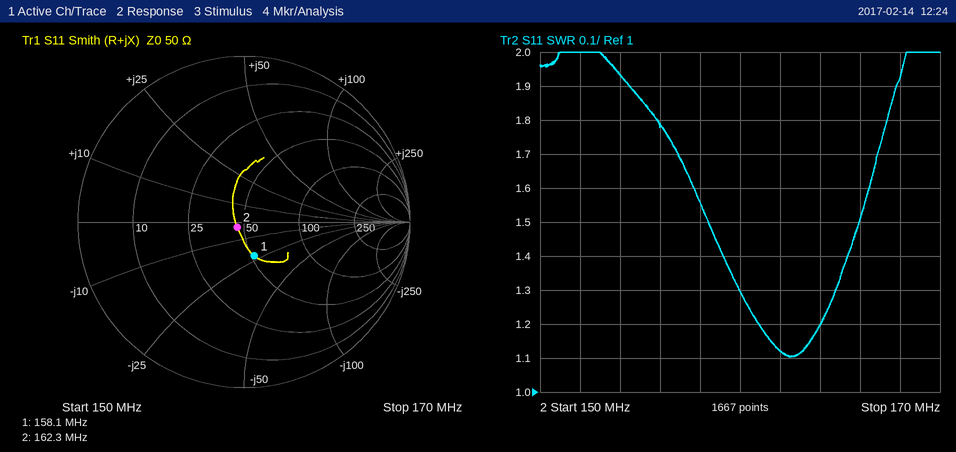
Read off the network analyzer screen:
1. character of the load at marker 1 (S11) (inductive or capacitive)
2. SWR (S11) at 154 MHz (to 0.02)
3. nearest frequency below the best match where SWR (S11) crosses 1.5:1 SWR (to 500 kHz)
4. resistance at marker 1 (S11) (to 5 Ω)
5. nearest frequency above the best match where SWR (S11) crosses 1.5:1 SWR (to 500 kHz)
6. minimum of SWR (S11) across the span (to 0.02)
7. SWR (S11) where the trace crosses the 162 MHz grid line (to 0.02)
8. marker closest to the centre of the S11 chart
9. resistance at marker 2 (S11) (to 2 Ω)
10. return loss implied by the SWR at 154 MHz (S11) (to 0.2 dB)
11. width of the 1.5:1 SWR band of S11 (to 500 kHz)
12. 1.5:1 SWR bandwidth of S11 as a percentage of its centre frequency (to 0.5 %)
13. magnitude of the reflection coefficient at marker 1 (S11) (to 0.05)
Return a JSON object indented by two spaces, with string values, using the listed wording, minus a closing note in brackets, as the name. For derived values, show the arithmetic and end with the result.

{
  "character of the load at marker 1 (S11)": "capacitive",
  "SWR (S11) at 154 MHz": "1.94",
  "nearest frequency below the best match where SWR (S11) crosses 1.5:1 SWR": "158.5 MHz",
  "resistance at marker 1 (S11)": "50 Ω",
  "nearest frequency above the best match where SWR (S11) crosses 1.5:1 SWR": "166.0 MHz",
  "minimum of SWR (S11) across the span": "1.10",
  "SWR (S11) where the trace crosses the 162 MHz grid line": "1.12",
  "marker closest to the centre of the S11 chart": "marker 2",
  "resistance at marker 2 (S11)": "46 Ω",
  "return loss implied by the SWR at 154 MHz (S11)": "−20 log10((1.94 − 1)/(1.94 + 1)) ≈ 9.90 dB, so 10.0 dB to the nearest 0.2 dB",
  "width of the 1.5:1 SWR band of S11": "166.0 MHz − 158.5 MHz = 7.5 MHz",
  "1.5:1 SWR bandwidth of S11 as a percentage of its centre frequency": "7.5 MHz / 162.25 MHz ≈ 4.62 %, so 4.5 % to the nearest 0.5 %",
  "magnitude of the reflection coefficient at marker 1 (S11)": "0.20"
}
